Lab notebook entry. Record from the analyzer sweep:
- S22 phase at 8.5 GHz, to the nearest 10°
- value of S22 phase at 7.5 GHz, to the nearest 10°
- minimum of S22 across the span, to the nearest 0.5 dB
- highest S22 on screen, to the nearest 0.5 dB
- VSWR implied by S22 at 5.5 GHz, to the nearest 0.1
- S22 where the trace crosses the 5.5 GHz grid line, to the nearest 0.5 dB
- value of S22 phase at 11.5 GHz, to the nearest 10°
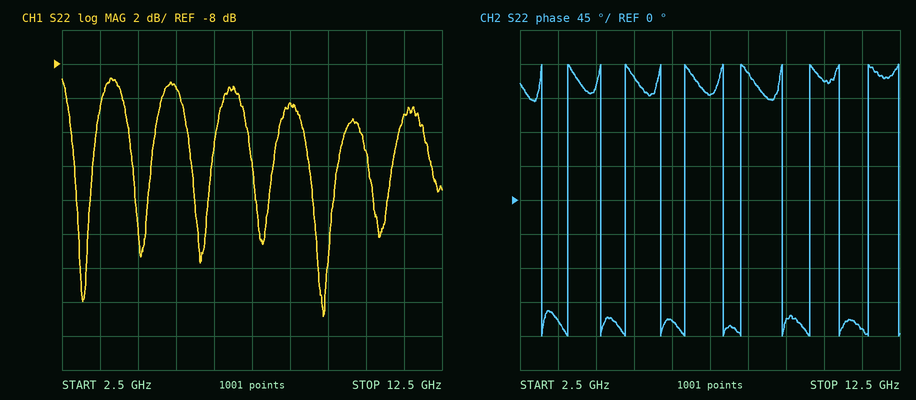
170°
140°
-23.0 dB
-9.0 dB
2.0
-9.5 dB
-170°
